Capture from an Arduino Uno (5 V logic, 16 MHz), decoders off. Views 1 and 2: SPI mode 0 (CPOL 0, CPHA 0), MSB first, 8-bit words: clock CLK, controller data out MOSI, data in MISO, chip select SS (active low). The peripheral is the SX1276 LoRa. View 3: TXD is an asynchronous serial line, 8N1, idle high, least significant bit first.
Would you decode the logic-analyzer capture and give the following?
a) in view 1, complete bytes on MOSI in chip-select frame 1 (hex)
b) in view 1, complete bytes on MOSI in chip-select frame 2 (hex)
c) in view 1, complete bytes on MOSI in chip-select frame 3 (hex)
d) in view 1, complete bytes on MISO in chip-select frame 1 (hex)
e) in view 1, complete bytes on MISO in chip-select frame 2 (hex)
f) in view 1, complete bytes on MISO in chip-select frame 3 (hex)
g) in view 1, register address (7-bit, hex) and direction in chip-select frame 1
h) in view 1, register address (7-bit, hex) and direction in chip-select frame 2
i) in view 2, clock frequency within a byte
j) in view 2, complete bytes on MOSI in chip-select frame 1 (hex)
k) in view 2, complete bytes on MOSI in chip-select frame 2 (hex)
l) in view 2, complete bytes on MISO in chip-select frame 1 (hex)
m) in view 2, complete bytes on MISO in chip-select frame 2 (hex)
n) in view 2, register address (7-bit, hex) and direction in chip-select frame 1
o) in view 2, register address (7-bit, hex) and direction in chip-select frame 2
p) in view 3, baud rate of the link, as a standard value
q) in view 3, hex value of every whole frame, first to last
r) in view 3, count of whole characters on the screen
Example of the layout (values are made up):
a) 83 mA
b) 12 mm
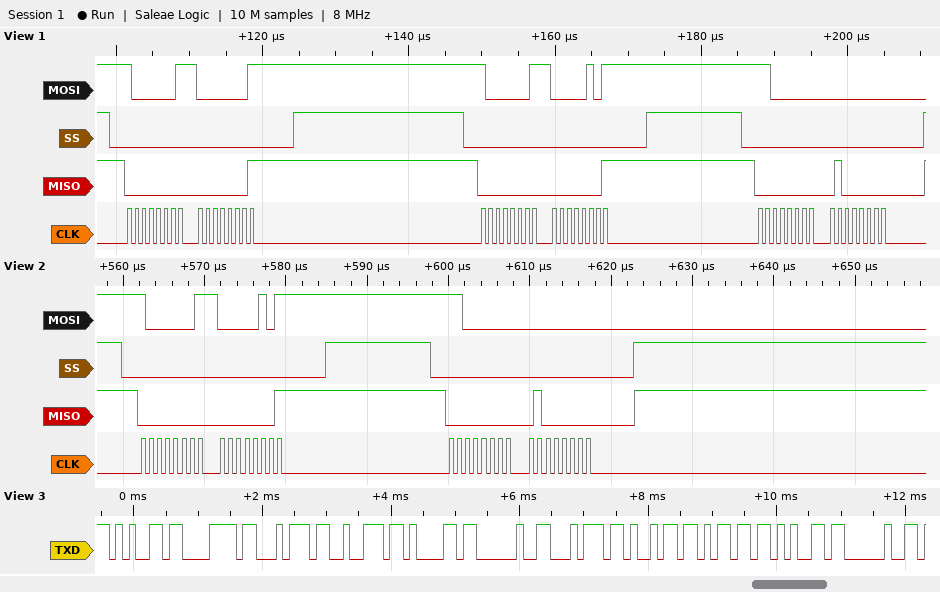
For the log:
a) 81 01
b) 81 05
c) C0 00
d) 00 01
e) 00 01
f) 00 40
g) 0x01 write
h) 0x01 write
i) 1 MHz
j) 81 05
k) C0 00
l) 00 01
m) 00 40
n) 0x01 write
o) 0x40 write
p) 9600 baud
q) 65 78 74 72 61 20 74 69 6D 65 20
r) 11
